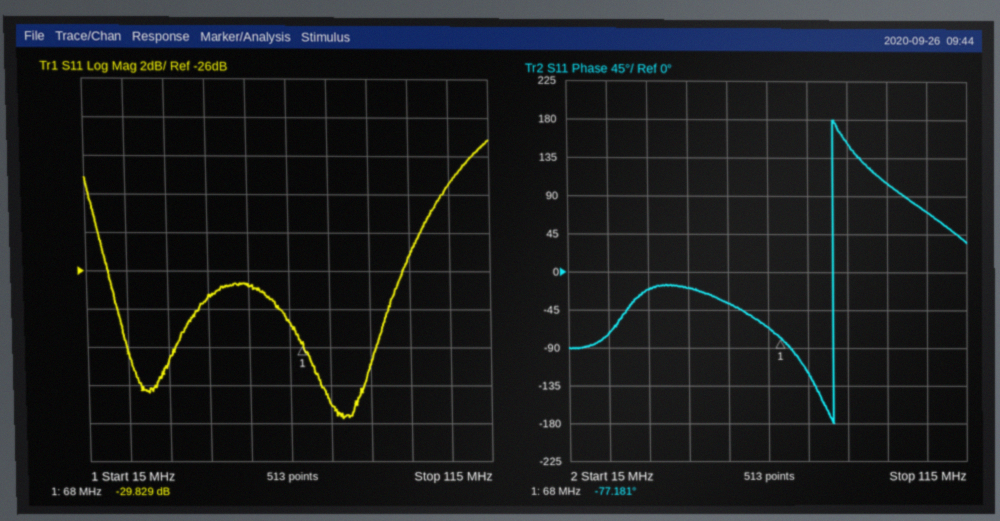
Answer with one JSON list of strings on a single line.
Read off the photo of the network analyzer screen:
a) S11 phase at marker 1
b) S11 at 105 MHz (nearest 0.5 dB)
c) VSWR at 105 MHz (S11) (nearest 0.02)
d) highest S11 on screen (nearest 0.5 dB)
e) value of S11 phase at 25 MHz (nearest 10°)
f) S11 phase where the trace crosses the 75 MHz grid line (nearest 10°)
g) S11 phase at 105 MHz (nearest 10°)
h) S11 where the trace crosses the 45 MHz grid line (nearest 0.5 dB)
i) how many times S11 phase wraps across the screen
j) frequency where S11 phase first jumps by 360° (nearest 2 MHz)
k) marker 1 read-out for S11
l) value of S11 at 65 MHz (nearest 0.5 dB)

["-77.181°", "-21.5 dB", "1.18", "-19.0 dB", "-70°", "-120°", "70°", "-27.5 dB", "1", "82 MHz", "-29.829 dB", "-28.5 dB"]
